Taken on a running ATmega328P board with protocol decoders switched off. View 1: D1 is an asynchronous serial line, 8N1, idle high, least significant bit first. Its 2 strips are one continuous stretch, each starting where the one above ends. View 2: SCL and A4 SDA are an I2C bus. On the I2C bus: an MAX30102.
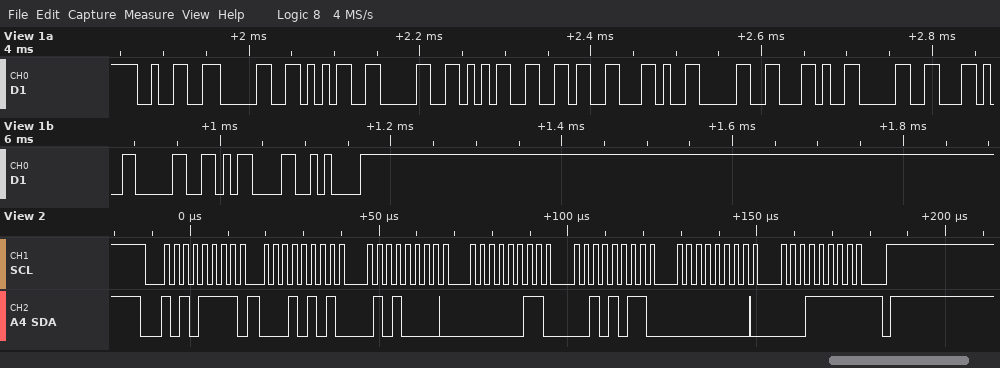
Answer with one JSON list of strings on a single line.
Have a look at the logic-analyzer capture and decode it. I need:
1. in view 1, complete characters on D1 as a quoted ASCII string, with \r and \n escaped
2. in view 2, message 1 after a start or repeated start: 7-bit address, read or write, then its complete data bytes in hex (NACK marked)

["\"205056,0,0,0\\r\\n\"", "0x57 read: 15 50 03 2B 00 1F NACK"]
